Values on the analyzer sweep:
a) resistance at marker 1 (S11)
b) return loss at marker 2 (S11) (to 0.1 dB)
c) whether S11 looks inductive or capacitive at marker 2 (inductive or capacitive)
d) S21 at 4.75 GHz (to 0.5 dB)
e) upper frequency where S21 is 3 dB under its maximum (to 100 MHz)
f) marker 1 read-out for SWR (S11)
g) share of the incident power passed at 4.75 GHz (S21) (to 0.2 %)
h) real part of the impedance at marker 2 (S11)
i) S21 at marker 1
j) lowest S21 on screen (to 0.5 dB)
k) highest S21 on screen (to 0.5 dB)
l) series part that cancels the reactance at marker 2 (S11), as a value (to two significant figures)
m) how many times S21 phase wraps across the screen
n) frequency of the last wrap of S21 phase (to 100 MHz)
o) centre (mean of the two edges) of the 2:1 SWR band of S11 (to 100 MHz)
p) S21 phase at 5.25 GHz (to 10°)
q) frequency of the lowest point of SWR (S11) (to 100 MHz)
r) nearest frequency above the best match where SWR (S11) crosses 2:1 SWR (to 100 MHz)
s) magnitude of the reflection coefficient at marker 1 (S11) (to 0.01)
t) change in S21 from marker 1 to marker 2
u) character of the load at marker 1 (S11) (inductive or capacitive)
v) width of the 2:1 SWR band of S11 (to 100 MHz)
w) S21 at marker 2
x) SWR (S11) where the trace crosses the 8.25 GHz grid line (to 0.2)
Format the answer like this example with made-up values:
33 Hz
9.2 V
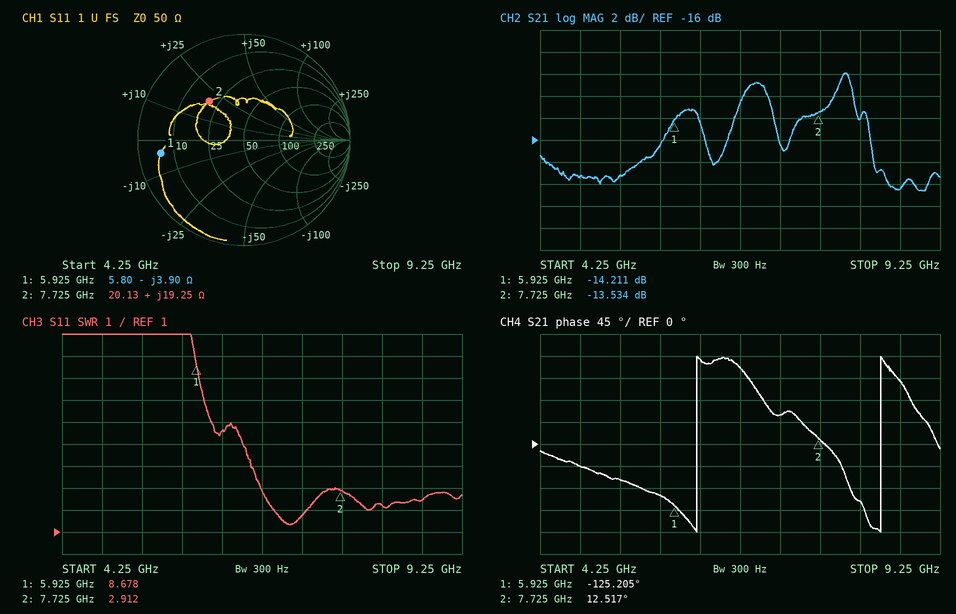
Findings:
5.80 Ω
6.2 dB
inductive
-19.5 dB
8.2 GHz
8.678
1.2 %
20.13 Ω
-14.211 dB
-20.5 dB
-10.0 dB
1.1 pF
2
8.5 GHz
7.1 GHz
-70°
7.1 GHz
7.3 GHz
0.79
0.677 dB
capacitive
400 MHz
-13.534 dB
2.2
